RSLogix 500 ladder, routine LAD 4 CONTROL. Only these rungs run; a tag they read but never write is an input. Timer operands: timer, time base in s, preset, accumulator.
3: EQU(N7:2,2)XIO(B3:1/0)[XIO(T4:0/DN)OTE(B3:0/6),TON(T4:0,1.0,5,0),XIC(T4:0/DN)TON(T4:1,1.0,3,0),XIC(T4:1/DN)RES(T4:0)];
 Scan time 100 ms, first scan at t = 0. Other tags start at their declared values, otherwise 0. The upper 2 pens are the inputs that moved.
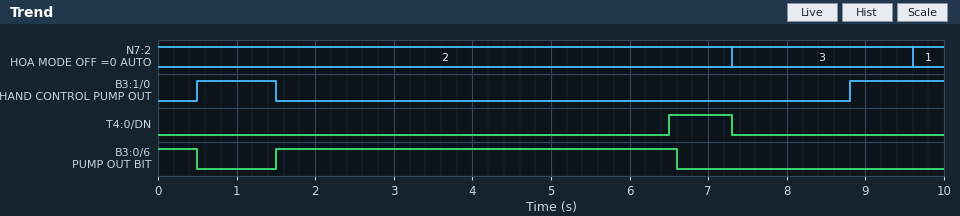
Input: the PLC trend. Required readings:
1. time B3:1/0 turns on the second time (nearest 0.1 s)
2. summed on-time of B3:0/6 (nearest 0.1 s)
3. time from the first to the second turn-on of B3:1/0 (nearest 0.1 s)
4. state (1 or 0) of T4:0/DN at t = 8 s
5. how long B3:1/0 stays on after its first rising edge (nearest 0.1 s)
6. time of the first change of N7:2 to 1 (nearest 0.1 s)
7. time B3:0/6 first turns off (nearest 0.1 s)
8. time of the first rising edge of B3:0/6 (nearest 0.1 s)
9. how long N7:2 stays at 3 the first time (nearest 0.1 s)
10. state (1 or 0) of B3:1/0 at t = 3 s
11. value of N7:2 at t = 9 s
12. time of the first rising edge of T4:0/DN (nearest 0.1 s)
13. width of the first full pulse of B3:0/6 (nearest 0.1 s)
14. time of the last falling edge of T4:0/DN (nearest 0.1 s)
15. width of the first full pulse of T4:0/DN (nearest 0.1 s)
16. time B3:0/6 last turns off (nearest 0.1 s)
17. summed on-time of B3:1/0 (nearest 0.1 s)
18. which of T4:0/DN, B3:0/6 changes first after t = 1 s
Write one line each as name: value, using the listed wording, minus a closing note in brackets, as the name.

time B3:1/0 turns on the second time: 8.8 s
summed on-time of B3:0/6: 5.6 s
time from the first to the second turn-on of B3:1/0: 8.3 s
state (1 or 0) of T4:0/DN at t = 8 s: 0
how long B3:1/0 stays on after its first rising edge: 1.0 s
time of the first change of N7:2 to 1: 9.6 s
time B3:0/6 first turns off: 0.5 s
time of the first rising edge of B3:0/6: 1.5 s
how long N7:2 stays at 3 the first time: 2.3 s
state (1 or 0) of B3:1/0 at t = 3 s: 0
value of N7:2 at t = 9 s: 3
time of the first rising edge of T4:0/DN: 6.5 s
width of the first full pulse of B3:0/6: 5.1 s
time of the last falling edge of T4:0/DN: 7.3 s
width of the first full pulse of T4:0/DN: 0.8 s
time B3:0/6 last turns off: 6.6 s
summed on-time of B3:1/0: 2.2 s
which of T4:0/DN, B3:0/6 changes first after t = 1 s: B3:0/6
